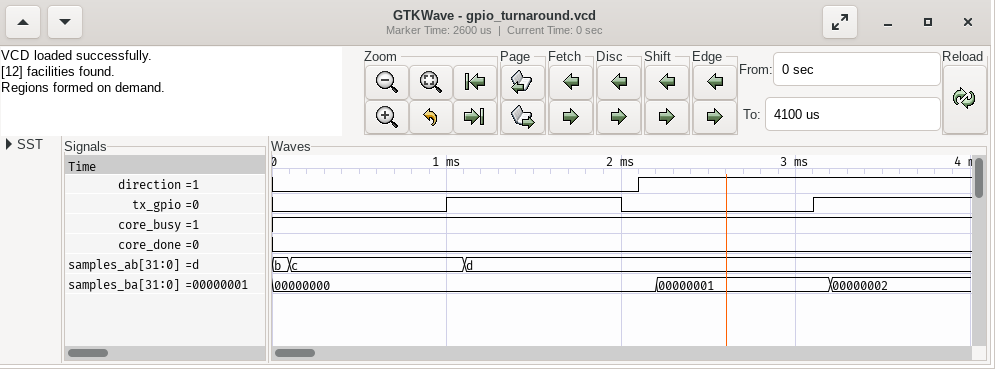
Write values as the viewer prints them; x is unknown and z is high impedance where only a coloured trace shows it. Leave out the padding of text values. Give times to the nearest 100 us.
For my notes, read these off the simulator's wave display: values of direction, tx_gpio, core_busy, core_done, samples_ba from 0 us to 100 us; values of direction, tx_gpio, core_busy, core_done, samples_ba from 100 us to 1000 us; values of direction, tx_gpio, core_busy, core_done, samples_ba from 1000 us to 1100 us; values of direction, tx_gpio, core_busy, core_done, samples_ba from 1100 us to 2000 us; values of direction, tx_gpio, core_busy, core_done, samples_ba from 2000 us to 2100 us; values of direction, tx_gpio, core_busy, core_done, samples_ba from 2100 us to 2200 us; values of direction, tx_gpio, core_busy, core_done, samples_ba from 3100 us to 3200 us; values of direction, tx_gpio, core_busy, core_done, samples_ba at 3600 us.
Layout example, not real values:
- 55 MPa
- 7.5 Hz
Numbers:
- direction=0, tx_gpio=0, core_busy=1, core_done=0, samples_ba=00000000
- direction=0, tx_gpio=0, core_busy=1, core_done=0, samples_ba=00000000
- direction=0, tx_gpio=1, core_busy=1, core_done=0, samples_ba=00000000
- direction=0, tx_gpio=1, core_busy=1, core_done=0, samples_ba=00000000
- direction=0, tx_gpio=0, core_busy=1, core_done=0, samples_ba=00000000
- direction=1, tx_gpio=0, core_busy=1, core_done=0, samples_ba=00000000
- direction=1, tx_gpio=1, core_busy=1, core_done=0, samples_ba=00000001
- direction=1, tx_gpio=1, core_busy=1, core_done=0, samples_ba=00000002
